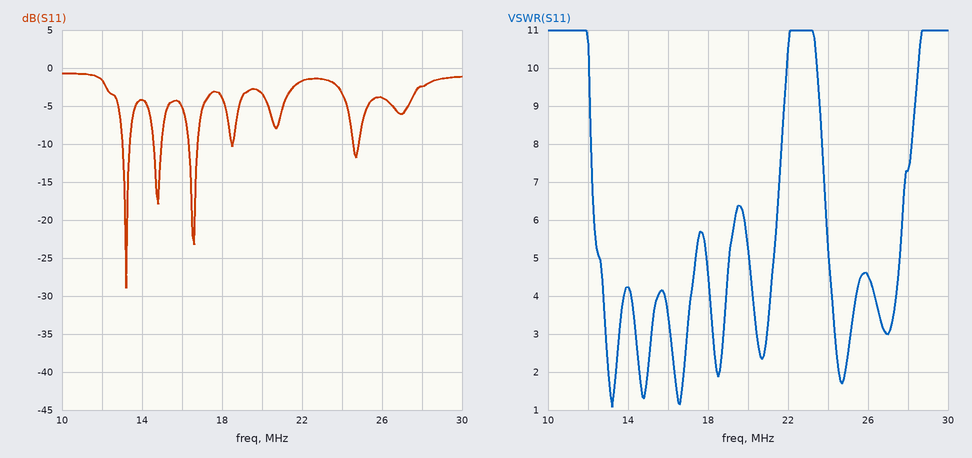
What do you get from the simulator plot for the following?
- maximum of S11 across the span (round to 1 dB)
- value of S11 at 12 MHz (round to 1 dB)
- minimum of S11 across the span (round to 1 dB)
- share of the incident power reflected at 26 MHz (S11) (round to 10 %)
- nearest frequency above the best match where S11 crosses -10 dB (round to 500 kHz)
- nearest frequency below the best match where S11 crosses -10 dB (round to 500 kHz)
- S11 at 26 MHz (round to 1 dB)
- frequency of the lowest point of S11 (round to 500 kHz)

-1 dB
-2 dB
-29 dB
40 %
13.5 MHz
13.0 MHz
-4 dB
13.0 MHz
